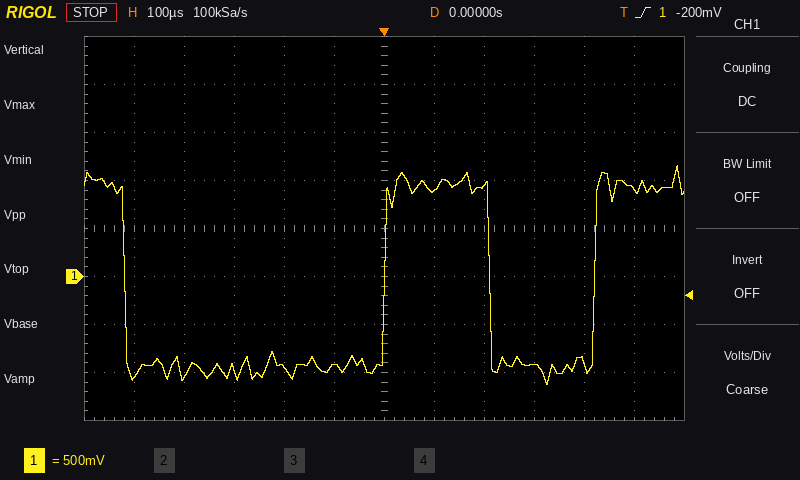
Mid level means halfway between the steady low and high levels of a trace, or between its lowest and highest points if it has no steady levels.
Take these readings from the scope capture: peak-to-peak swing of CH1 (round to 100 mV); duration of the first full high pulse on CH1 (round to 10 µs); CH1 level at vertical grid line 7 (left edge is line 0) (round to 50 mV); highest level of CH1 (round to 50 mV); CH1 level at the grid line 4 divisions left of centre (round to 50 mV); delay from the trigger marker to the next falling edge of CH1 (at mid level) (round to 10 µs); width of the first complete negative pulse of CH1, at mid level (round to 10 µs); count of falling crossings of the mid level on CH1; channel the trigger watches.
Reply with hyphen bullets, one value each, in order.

- 2.30 V
- 210 µs
- 900 mV
- 1.15 V
- -1.05 V
- 210 µs
- 520 µs
- 2
- CH1
